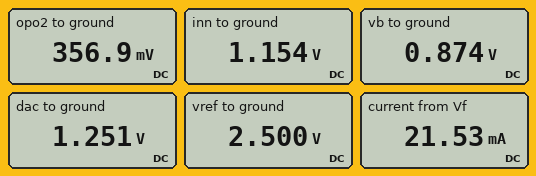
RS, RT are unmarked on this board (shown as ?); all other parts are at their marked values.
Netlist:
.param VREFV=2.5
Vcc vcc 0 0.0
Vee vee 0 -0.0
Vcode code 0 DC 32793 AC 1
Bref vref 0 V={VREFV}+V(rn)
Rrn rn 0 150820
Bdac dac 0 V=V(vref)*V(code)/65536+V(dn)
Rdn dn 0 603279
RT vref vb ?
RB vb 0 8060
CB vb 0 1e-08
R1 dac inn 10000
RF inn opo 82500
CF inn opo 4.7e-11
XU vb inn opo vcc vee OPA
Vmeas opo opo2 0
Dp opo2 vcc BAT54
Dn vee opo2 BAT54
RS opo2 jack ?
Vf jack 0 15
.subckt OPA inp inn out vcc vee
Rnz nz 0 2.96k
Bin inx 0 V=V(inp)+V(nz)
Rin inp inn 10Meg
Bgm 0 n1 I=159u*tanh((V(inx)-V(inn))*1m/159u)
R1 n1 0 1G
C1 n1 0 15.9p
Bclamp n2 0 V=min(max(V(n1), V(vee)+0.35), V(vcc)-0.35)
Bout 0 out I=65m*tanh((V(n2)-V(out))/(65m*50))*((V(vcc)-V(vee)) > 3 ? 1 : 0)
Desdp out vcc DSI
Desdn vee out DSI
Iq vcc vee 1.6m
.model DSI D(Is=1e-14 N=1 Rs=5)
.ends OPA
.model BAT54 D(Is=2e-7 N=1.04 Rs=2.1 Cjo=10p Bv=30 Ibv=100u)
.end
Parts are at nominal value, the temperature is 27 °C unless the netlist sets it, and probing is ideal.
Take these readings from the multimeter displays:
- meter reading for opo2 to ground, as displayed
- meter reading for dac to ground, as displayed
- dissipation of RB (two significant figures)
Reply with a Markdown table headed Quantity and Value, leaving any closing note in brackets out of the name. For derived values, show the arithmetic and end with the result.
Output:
| Quantity | Value |
|---|---|
| meter reading for opo2 to ground, as displayed | 356.9 mV |
| meter reading for dac to ground, as displayed | 1.251 V |
| dissipation of RB | (874 mV)^2 / 8.06 kΩ = 95 µW |
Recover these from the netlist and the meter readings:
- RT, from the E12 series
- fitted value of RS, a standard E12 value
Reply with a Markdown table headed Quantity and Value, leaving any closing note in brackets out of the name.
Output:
| Quantity | Value |
|---|---|
| RT, from the E12 series | 15 kΩ |
| fitted value of RS, a standard E12 value | 680 Ω |
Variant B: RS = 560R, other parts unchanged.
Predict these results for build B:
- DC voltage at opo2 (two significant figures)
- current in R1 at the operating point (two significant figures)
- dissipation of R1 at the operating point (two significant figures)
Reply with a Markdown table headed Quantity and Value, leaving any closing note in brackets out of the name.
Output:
| Quantity | Value |
|---|---|
| DC voltage at opo2 | 370 mV |
| current in R1 at the operating point | 9.5 µA |
| dissipation of R1 at the operating point | 910 nW |
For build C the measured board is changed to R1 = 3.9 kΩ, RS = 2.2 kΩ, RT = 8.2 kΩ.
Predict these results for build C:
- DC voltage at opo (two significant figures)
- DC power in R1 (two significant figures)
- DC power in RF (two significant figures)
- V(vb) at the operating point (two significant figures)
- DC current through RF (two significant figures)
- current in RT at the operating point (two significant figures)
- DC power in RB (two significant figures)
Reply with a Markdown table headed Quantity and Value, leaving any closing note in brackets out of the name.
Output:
| Quantity | Value |
|---|---|
| DC voltage at opo | 290 mV |
| DC power in R1 | 480 nW |
| DC power in RF | 10 µW |
| V(vb) at the operating point | 1.2 V |
| DC current through RF | 11 µA |
| current in RT at the operating point | 150 µA |
| DC power in RB | 190 µW |
